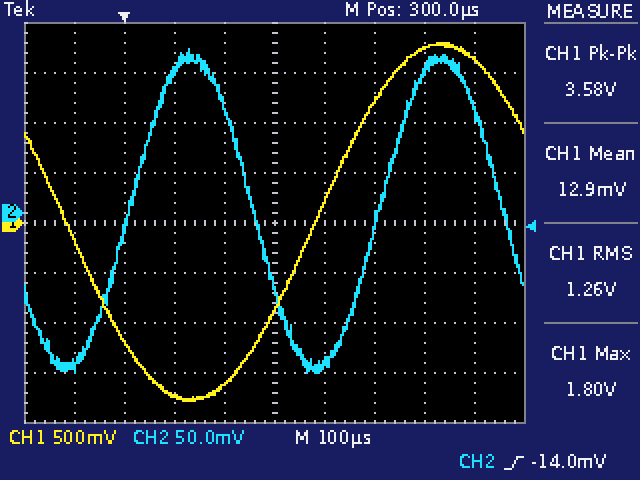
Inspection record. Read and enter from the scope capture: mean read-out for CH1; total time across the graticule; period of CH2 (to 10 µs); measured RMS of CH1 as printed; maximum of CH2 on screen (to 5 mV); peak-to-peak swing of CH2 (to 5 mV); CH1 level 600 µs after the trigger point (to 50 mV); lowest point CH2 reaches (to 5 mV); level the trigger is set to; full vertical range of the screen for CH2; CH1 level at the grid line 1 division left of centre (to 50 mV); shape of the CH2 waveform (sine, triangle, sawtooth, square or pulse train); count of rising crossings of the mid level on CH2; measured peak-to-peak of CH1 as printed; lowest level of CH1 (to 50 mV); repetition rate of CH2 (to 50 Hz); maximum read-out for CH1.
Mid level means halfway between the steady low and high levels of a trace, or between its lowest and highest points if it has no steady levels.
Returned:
12.9 mV
1 ms
500 µs
1.26 V
165 mV
325 mV
1.75 V
-160 mV
-14.0 mV
400 mV
-1.60 V
sine
2
3.58 V
-1.80 V
2.00 kHz
1.80 V
